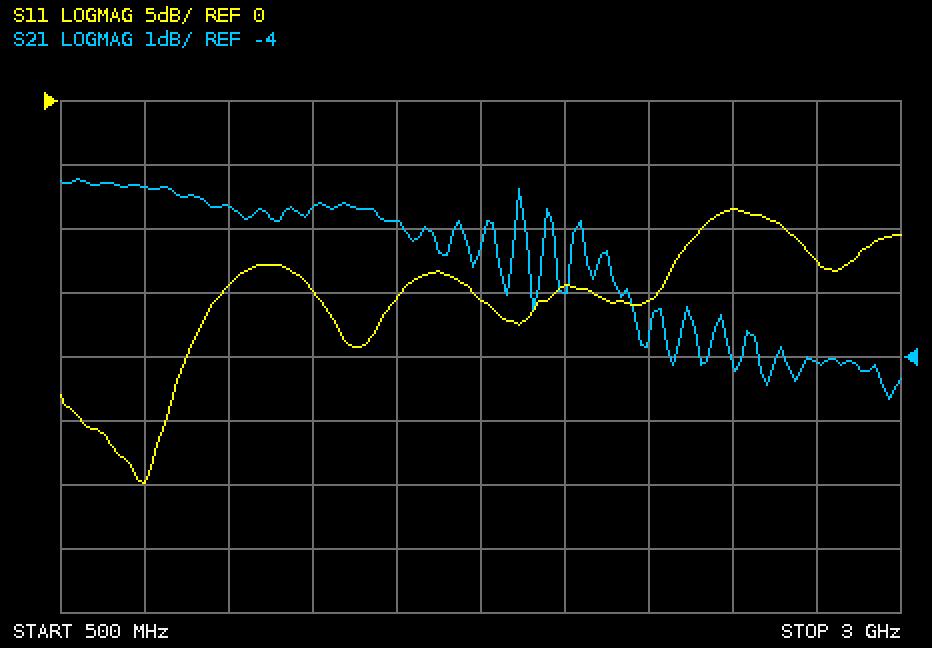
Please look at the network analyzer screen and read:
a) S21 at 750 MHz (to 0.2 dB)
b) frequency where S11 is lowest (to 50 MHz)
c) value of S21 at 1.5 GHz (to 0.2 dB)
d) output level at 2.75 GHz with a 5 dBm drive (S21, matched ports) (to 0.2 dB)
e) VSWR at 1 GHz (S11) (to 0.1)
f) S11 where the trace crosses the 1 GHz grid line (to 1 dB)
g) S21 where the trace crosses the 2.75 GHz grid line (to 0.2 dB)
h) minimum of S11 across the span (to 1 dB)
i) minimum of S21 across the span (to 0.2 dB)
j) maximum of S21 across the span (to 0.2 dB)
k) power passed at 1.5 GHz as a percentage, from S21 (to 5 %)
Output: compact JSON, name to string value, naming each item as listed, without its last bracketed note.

{"S21 at 750 MHz": "-1.4 dB", "frequency where S11 is lowest": "750 MHz", "value of S21 at 1.5 GHz": "-1.8 dB", "output level at 2.75 GHz with a 5 dBm drive (S21, matched ports)": "1.0 dBm", "VSWR at 1 GHz (S11)": "1.5", "S11 where the trace crosses the 1 GHz grid line": "-14 dB", "S21 where the trace crosses the 2.75 GHz grid line": "-4.0 dB", "minimum of S11 across the span": "-30 dB", "minimum of S21 across the span": "-4.6 dB", "maximum of S21 across the span": "-1.2 dB", "power passed at 1.5 GHz as a percentage, from S21": "65 %"}
